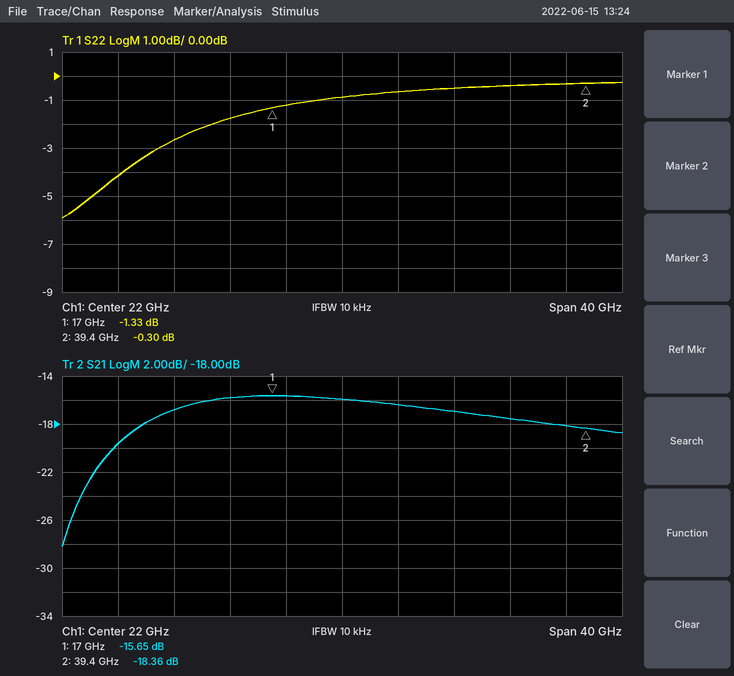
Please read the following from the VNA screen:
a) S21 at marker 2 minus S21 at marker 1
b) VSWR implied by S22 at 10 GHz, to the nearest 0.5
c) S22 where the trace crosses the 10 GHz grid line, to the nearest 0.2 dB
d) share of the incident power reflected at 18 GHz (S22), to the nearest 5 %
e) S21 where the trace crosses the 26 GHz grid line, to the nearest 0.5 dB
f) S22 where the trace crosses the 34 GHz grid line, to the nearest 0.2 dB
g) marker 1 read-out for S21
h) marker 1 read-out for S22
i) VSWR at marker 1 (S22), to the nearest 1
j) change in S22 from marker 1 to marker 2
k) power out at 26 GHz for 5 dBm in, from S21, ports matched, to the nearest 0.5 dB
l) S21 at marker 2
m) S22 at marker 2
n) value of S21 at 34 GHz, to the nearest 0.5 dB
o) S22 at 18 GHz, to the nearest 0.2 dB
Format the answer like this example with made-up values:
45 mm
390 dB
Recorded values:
-2.71 dB
6.5
-2.6 dB
75 %
-16.5 dB
-0.4 dB
-15.65 dB
-1.33 dB
13
1.03 dB
-11.5 dBm
-18.36 dB
-0.30 dB
-17.5 dB
-1.2 dB
